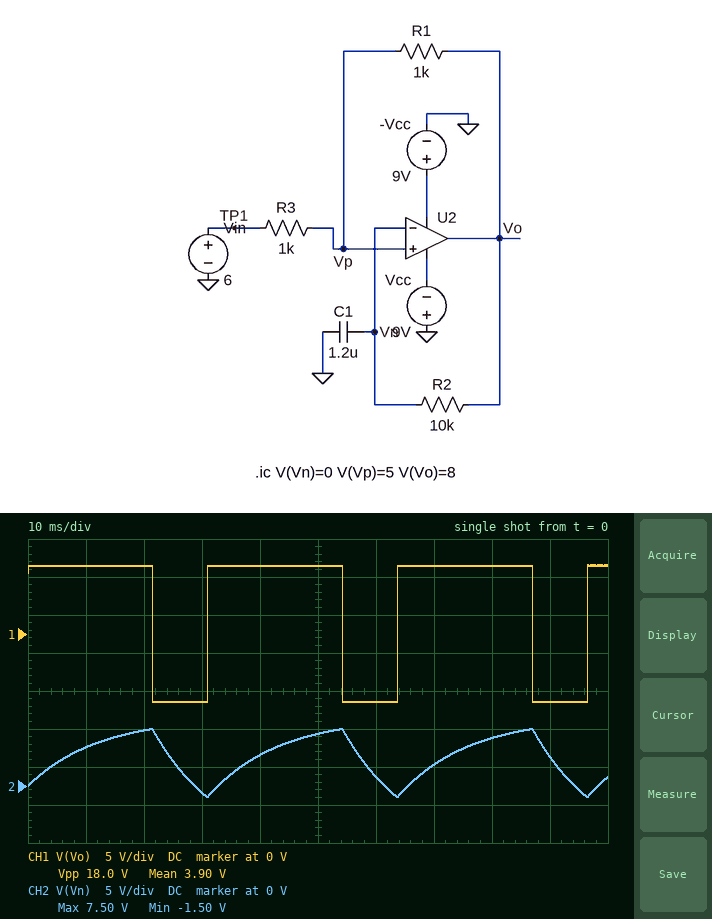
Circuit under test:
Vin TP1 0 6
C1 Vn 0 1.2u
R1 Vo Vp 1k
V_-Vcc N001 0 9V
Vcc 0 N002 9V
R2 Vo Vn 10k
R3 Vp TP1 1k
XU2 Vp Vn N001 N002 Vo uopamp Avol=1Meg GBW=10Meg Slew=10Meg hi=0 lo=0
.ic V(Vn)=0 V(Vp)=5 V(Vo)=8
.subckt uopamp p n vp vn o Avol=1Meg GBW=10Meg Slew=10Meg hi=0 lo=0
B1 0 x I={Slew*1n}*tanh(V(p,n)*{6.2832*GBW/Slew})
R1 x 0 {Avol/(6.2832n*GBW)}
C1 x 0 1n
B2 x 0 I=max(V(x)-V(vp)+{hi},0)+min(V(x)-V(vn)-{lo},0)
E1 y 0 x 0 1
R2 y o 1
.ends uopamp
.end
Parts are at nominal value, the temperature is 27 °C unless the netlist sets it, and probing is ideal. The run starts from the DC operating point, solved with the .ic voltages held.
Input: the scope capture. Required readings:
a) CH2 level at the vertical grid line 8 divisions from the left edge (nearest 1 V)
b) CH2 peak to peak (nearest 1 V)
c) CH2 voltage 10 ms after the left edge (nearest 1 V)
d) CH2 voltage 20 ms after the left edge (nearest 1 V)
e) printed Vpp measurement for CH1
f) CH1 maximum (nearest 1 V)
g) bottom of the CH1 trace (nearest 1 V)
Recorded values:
6 V
9 V
5 V
7 V
18.0 V
9 V
-9 V
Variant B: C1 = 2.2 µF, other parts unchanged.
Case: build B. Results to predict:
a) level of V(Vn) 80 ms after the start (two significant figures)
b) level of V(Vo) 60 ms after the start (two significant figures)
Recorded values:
5.4 V
9.0 V
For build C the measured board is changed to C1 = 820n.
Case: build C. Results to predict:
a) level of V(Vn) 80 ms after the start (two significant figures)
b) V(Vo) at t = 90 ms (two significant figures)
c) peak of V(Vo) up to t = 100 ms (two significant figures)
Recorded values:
7.1 V
9.0 V
9.0 V
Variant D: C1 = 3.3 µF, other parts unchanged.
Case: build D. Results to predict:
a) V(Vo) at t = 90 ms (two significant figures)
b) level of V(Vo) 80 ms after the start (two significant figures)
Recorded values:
9.0 V
-9.0 V
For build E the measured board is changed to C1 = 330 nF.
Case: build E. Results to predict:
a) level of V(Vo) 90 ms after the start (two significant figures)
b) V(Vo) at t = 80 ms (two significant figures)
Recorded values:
9.0 V
-9.0 V
